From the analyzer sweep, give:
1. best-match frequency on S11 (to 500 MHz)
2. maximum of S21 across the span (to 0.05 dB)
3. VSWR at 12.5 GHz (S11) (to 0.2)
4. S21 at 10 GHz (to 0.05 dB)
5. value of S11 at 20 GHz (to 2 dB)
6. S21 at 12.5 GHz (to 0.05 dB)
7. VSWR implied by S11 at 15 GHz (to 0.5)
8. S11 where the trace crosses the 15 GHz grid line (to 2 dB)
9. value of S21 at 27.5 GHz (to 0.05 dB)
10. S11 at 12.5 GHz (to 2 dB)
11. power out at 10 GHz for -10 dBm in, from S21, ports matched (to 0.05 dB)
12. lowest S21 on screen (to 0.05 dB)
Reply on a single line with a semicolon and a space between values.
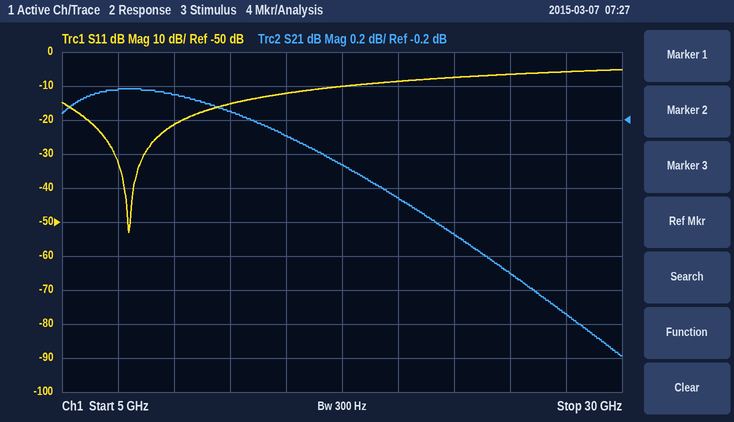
8.0 GHz; 0.00 dB; 1.4; -0.05 dB; -8 dB; -0.15 dB; 1.5; -12 dB; -1.35 dB; -16 dB; -10.05 dBm; -1.60 dB
